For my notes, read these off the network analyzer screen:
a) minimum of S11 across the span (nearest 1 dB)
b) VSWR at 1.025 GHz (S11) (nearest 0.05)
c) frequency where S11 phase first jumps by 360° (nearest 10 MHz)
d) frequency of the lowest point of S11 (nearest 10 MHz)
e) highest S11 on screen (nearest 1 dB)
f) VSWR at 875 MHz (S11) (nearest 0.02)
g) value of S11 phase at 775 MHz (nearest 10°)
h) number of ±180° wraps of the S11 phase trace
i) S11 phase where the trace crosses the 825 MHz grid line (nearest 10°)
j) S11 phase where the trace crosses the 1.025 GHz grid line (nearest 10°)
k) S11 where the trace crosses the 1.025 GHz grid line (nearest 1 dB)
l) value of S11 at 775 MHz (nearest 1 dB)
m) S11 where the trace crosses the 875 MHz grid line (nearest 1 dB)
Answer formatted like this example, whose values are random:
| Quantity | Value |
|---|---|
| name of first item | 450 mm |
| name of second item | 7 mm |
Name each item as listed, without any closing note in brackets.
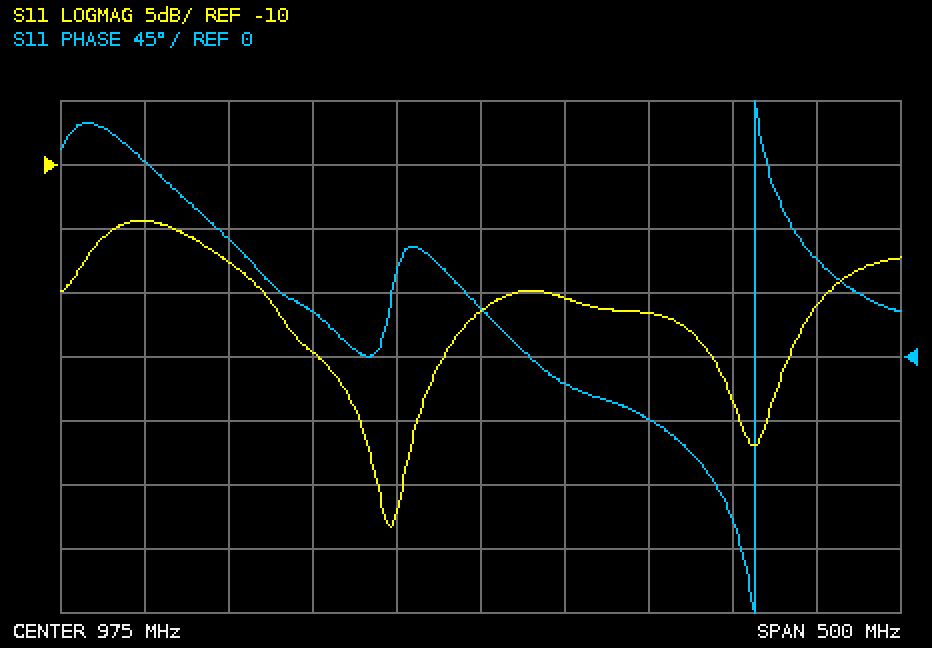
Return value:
| Quantity | Value |
|---|---|
| minimum of S11 across the span | -38 dB |
| VSWR at 1.025 GHz (S11) | 1.20 |
| frequency where S11 phase first jumps by 360° | 1.14 GHz |
| frequency of the lowest point of S11 | 920 MHz |
| highest S11 on screen | -14 dB |
| VSWR at 875 MHz (S11) | 1.12 |
| value of S11 phase at 775 MHz | 140° |
| number of ±180° wraps of the S11 phase trace | 1 |
| S11 phase where the trace crosses the 825 MHz grid line | 80° |
| S11 phase where the trace crosses the 1.025 GHz grid line | -20° |
| S11 where the trace crosses the 1.025 GHz grid line | -20 dB |
| value of S11 at 775 MHz | -14 dB |
| S11 where the trace crosses the 875 MHz grid line | -25 dB |
